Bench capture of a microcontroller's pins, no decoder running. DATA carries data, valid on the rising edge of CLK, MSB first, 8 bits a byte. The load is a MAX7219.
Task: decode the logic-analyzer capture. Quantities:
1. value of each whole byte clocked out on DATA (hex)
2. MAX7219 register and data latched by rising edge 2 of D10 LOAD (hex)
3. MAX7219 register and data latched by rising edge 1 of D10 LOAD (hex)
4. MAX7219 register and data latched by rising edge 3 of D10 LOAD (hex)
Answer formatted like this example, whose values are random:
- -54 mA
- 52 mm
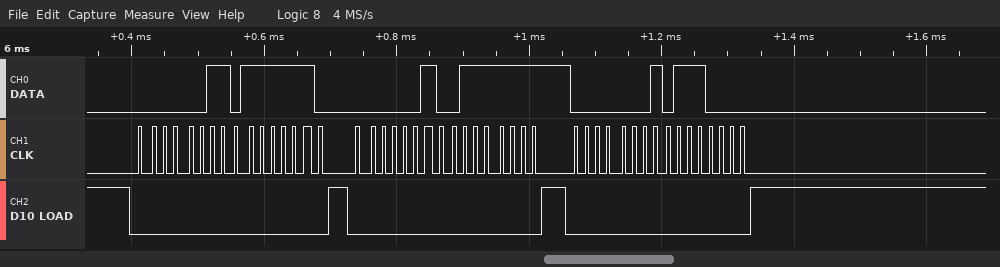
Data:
- 0x03 0x7E 0x02 0x7F 0x01 0x70
- register 0x2, data 0x7F
- register 0x3, data 0x7E
- register 0x1, data 0x70
